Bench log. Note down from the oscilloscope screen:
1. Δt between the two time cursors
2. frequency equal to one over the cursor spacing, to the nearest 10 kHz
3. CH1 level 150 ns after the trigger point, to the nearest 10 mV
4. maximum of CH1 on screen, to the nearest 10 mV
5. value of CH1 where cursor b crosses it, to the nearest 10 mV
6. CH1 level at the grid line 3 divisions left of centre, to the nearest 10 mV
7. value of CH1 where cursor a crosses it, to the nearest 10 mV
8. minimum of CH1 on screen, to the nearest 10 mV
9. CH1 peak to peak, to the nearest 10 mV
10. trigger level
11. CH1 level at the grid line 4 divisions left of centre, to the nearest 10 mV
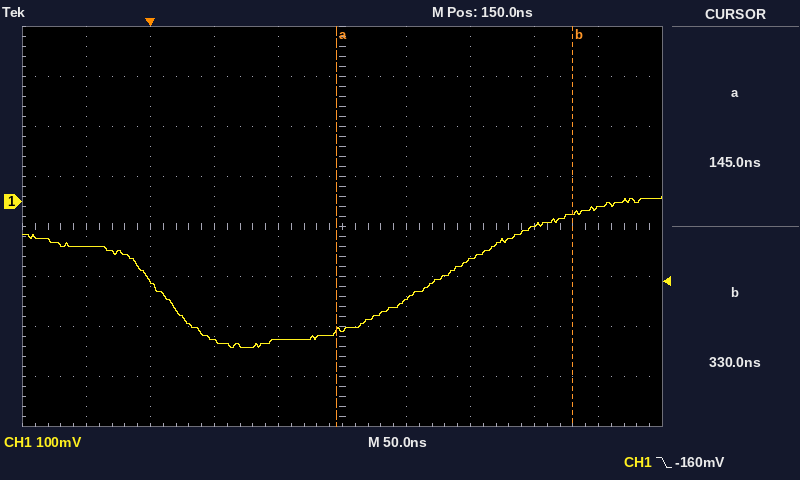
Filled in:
185 ns
5.41 MHz
-260 mV
10 mV
-20 mV
-160 mV
-260 mV
-290 mV
300 mV
-160 mV
-90 mV
